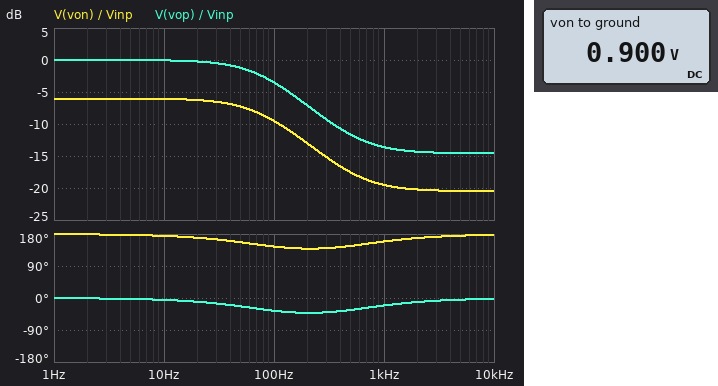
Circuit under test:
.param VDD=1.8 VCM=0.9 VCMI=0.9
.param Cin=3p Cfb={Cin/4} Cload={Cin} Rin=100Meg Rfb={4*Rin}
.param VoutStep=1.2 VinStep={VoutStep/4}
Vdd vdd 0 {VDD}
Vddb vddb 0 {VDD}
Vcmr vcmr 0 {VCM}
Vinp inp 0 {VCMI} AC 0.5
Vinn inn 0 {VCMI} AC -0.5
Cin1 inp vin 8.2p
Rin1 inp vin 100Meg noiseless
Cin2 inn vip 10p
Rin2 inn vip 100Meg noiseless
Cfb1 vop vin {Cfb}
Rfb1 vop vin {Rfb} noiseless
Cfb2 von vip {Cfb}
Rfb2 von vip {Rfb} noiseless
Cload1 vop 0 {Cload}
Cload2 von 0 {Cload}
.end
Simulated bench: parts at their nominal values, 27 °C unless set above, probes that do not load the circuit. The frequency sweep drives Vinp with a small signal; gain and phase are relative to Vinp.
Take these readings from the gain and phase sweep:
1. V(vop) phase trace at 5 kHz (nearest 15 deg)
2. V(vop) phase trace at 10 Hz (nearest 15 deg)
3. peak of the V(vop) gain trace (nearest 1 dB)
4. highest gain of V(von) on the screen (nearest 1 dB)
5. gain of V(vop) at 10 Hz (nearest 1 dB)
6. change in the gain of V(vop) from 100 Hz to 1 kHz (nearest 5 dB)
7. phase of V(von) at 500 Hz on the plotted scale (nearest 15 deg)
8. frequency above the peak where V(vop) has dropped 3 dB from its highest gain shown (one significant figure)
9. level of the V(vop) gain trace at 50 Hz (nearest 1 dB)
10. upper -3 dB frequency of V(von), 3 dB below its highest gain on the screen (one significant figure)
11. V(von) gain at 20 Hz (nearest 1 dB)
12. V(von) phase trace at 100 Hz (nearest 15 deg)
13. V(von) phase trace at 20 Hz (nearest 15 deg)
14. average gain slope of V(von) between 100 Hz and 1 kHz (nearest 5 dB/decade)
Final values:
0 deg
0 deg
0 dB
-6 dB
0 dB
-10 dB
150 deg
90 Hz
-1 dB
90 Hz
-6 dB
150 deg
165 deg
-10 dB/decade
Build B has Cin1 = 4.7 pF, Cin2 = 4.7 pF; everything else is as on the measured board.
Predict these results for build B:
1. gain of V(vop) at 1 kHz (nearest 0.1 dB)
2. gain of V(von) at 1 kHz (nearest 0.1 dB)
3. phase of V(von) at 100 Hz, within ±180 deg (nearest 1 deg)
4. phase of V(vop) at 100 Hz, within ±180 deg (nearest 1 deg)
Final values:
-14.1 dB
-20.1 dB
143 deg
-37 deg
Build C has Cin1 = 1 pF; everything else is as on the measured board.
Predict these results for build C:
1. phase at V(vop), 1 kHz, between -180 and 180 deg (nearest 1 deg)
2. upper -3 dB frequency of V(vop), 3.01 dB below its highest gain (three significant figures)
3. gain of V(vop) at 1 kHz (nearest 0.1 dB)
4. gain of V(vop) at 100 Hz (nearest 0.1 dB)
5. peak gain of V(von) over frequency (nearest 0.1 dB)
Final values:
-31 deg
92.7 Hz
-15.3 dB
-3.3 dB
-6.0 dB
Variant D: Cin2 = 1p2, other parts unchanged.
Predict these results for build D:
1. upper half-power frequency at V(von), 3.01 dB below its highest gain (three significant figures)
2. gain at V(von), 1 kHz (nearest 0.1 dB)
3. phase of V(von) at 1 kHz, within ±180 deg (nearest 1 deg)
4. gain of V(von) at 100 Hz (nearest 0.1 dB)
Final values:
92.5 Hz
-21.3 dB
150 deg
-9.4 dB
